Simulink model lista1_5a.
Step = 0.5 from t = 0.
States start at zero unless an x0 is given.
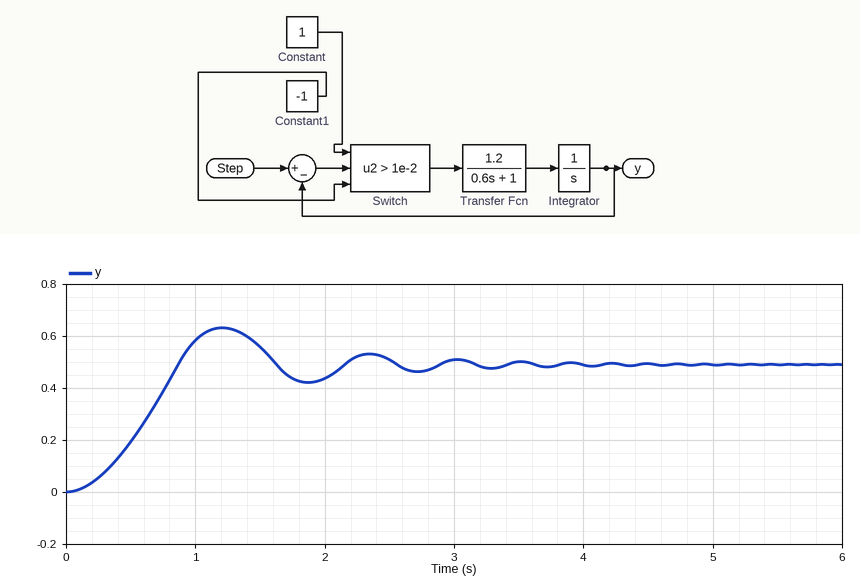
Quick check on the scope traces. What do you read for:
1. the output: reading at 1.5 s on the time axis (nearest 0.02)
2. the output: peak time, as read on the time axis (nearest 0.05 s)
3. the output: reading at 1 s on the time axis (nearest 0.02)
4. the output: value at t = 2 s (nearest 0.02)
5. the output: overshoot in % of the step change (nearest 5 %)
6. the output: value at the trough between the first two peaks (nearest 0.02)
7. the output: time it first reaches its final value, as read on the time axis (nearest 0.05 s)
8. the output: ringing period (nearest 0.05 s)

0.56
1.20 s
0.58
0.44
30 %
0.42
0.85 s
1.15 s
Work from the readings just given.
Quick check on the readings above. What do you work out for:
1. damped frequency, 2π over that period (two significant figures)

5.5 rad/s
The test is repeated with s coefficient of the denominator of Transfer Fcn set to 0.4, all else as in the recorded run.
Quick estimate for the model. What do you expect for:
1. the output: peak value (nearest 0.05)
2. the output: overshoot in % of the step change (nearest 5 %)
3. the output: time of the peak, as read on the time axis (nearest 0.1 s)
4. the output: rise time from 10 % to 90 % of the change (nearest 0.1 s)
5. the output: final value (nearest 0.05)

0.60
25 %
1.0 s
0.5 s
0.50
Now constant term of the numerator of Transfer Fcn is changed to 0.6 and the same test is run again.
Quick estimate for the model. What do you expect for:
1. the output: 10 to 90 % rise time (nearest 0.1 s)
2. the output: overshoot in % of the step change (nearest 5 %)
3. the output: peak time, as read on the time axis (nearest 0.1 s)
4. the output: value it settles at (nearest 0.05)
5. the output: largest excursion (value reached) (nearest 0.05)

0.9 s
20 %
1.7 s
0.50
0.60
